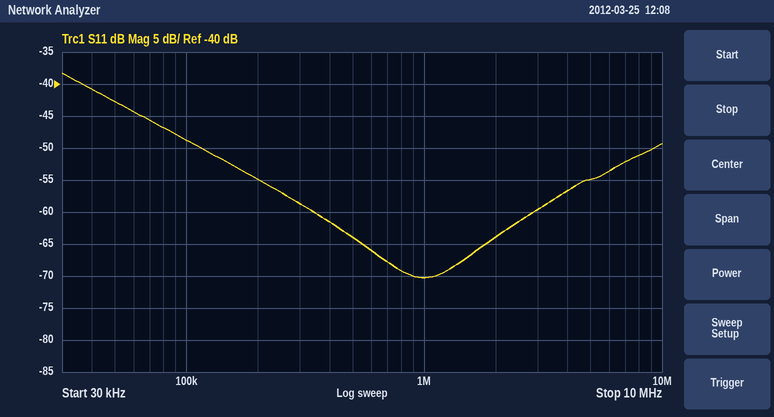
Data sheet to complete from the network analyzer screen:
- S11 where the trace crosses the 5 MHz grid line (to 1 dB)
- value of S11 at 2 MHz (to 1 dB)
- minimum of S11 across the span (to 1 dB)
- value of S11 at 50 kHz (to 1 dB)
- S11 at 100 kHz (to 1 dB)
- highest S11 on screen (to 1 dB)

-55 dB
-64 dB
-70 dB
-43 dB
-49 dB
-38 dB
